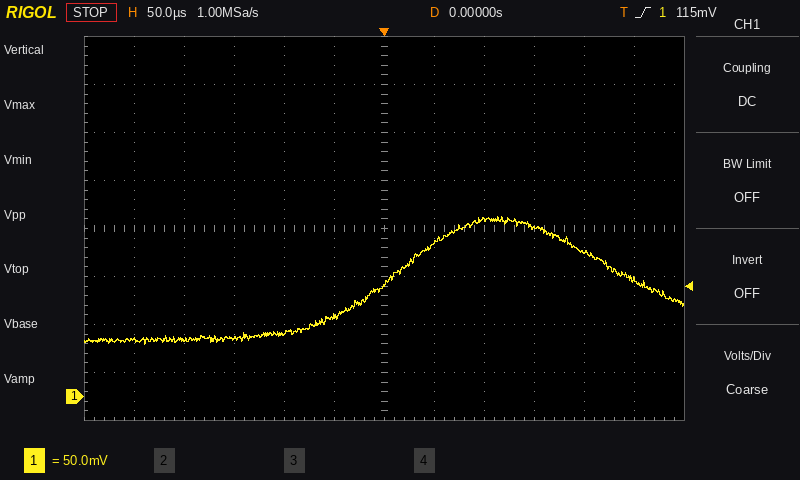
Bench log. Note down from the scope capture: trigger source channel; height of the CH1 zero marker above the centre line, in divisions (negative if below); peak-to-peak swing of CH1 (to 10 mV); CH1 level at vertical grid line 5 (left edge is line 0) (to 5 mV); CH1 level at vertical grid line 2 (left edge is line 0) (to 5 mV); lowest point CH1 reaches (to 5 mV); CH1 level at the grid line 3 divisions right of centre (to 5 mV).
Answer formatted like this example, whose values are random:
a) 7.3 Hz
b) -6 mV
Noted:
a) CH1
b) -3.5 div
c) 130 mV
d) 85 mV
e) 60 mV
f) 55 mV
g) 175 mV
